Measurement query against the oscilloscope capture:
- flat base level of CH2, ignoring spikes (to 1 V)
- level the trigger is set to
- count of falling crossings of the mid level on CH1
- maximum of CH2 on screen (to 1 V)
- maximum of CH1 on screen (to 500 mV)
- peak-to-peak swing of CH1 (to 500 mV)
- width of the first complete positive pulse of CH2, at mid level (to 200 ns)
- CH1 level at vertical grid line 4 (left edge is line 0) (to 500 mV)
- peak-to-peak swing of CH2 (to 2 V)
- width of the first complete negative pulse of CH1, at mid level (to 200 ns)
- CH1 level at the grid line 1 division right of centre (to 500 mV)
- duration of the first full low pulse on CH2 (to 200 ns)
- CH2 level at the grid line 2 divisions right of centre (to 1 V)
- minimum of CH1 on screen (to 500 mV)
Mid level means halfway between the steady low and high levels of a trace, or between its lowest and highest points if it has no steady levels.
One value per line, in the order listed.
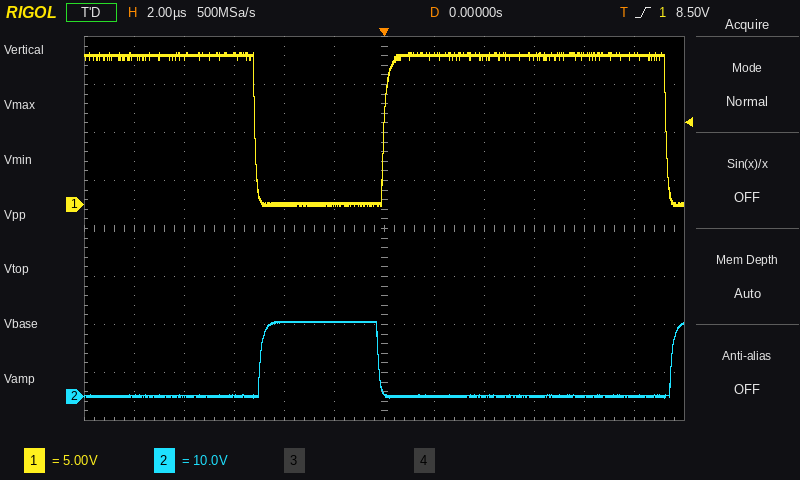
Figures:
0 V
8.50 V
2
16 V
16.0 V
16.0 V
4.8 µs
0.0 V
16 V
5.2 µs
15.5 V
11.8 µs
0 V
0.0 V
